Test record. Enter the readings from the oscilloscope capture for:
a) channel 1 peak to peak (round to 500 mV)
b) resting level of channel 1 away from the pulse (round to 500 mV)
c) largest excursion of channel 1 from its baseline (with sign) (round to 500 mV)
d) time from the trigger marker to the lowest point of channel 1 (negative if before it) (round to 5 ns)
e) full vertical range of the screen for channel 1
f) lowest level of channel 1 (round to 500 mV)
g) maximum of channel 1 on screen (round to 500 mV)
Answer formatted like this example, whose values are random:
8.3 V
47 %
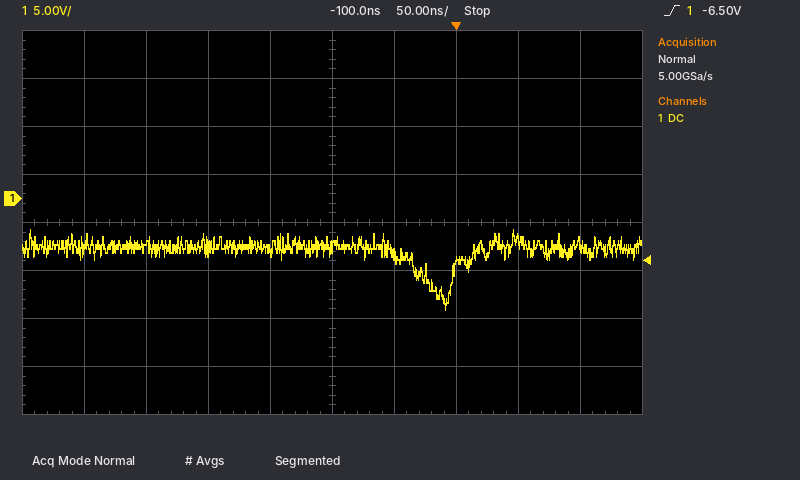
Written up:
8.5 V
-5.0 V
-6.5 V
-10 ns
40 V
-11.5 V
-3.0 V
